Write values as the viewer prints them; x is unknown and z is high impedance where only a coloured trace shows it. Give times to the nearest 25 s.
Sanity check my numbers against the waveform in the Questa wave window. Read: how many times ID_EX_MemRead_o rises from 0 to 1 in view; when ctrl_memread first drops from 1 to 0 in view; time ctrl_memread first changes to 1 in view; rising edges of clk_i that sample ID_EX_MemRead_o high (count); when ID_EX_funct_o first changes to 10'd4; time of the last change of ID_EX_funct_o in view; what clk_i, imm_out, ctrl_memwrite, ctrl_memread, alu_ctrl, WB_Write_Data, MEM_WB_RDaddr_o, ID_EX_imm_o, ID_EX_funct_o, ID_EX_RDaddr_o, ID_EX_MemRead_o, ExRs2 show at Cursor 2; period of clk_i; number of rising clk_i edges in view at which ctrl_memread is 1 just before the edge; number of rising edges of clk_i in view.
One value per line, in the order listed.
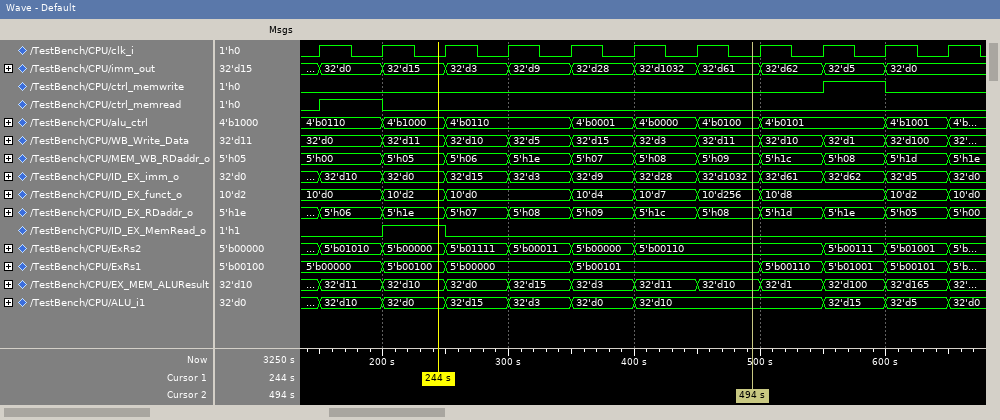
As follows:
1
200 s
150 s
1
350 s
650 s
clk_i=0, imm_out=32'd61, ctrl_memwrite=0, ctrl_memread=0, alu_ctrl=4'b0100, WB_Write_Data=32'd11, MEM_WB_RDaddr_o=5'h09, ID_EX_imm_o=32'd1032, ID_EX_funct_o=10'd256, ID_EX_RDaddr_o=5'h08, ID_EX_MemRead_o=0, ExRs2=5'b00110
50 s
1
11
